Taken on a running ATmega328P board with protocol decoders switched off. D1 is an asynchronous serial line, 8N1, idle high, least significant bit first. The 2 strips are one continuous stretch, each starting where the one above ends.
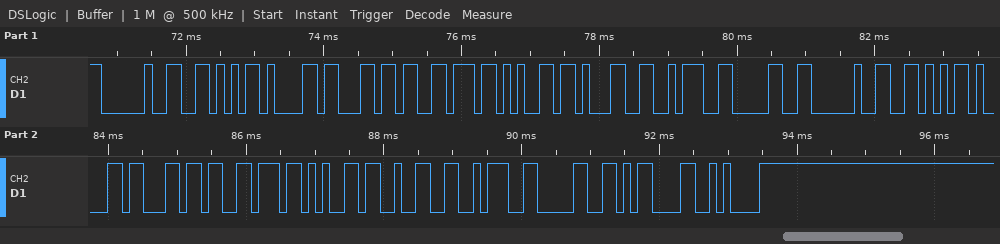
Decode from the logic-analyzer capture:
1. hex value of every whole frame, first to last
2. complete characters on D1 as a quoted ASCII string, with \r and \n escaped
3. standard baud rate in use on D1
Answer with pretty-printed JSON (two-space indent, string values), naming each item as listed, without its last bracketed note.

{
  "hex value of every whole frame, first to last": "20 56 61 6C 76 65 31 3A 30 20 56 61 6C 76 65 32 3A 30 0D 0A",
  "complete characters on D1 as a quoted ASCII string, with \\r and \\n escaped": "\" Valve1:0 Valve2:0\\r\\n\"",
  "standard baud rate in use on D1": "9600 baud"
}
